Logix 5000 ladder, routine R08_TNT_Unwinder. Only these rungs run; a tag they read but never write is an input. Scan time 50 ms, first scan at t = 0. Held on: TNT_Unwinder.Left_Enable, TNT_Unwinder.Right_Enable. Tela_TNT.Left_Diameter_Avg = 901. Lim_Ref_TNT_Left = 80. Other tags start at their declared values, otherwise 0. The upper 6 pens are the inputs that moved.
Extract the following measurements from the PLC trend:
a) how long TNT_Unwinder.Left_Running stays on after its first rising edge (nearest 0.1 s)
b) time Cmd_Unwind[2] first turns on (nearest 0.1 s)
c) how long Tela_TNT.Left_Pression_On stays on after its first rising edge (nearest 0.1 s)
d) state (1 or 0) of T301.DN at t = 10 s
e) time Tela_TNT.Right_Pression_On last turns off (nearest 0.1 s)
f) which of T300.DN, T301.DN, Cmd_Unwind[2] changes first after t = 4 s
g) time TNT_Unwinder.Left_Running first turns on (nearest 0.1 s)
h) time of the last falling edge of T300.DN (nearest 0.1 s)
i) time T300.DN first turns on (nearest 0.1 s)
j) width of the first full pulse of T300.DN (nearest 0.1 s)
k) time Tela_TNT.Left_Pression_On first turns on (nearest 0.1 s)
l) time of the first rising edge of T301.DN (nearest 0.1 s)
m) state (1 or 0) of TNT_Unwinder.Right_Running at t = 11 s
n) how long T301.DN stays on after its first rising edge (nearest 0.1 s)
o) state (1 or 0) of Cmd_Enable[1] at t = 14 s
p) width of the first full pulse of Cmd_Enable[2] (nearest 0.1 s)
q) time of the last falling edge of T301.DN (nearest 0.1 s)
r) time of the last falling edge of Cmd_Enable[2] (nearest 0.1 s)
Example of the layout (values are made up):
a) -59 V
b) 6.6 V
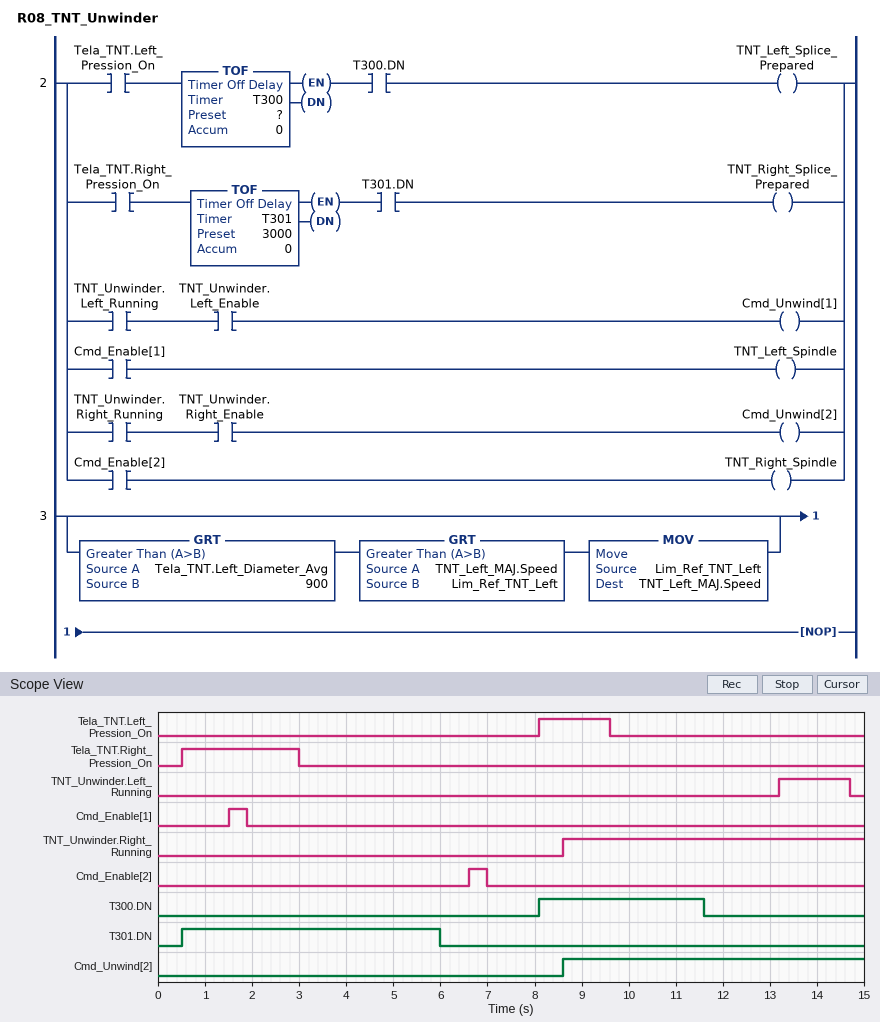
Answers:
a) 1.5 s
b) 8.6 s
c) 1.5 s
d) 0
e) 3.0 s
f) T301.DN
g) 13.2 s
h) 11.6 s
i) 8.1 s
j) 3.5 s
k) 8.1 s
l) 0.5 s
m) 1
n) 5.5 s
o) 0
p) 0.4 s
q) 6.0 s
r) 7.0 s
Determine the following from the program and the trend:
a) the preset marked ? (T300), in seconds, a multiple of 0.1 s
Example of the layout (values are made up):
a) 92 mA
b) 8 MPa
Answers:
a) 2.0 s
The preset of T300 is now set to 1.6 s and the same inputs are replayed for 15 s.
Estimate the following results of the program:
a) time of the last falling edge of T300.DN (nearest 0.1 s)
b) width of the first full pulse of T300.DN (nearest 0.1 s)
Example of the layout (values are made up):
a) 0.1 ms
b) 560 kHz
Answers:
a) 11.2 s
b) 3.1 s
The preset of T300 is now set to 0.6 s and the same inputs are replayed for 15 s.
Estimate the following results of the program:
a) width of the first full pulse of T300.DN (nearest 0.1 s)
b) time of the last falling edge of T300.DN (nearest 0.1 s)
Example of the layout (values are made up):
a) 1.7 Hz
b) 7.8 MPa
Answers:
a) 2.1 s
b) 10.2 s
